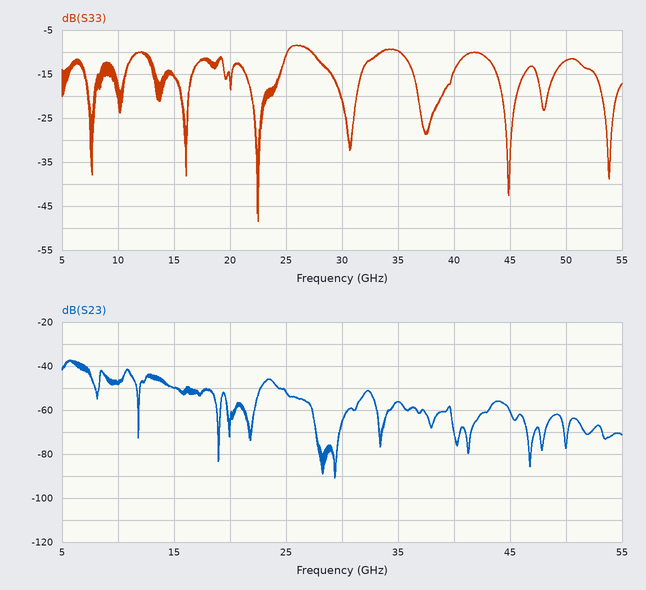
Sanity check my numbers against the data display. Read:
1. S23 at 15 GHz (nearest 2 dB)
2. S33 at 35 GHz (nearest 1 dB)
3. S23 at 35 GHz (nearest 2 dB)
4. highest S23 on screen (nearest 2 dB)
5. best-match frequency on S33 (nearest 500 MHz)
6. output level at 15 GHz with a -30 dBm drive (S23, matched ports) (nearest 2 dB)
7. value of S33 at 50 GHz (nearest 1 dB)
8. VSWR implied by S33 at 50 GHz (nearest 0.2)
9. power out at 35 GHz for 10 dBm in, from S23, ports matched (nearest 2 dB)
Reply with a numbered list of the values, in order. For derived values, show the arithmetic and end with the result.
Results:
1. -50 dB
2. -10 dB
3. -56 dB
4. -38 dB
5. 22.5 GHz
6. -30 dBm + (-50 dB) = -80 dBm
7. -12 dB
8. |Γ| = 10^(-12/20) = 0.2512; VSWR = (1 + 0.2512)/(1 − 0.2512) ≈ 1.67, so 1.6 to the nearest 0.2
9. 10 dBm + (-56 dB) = -46 dBm
